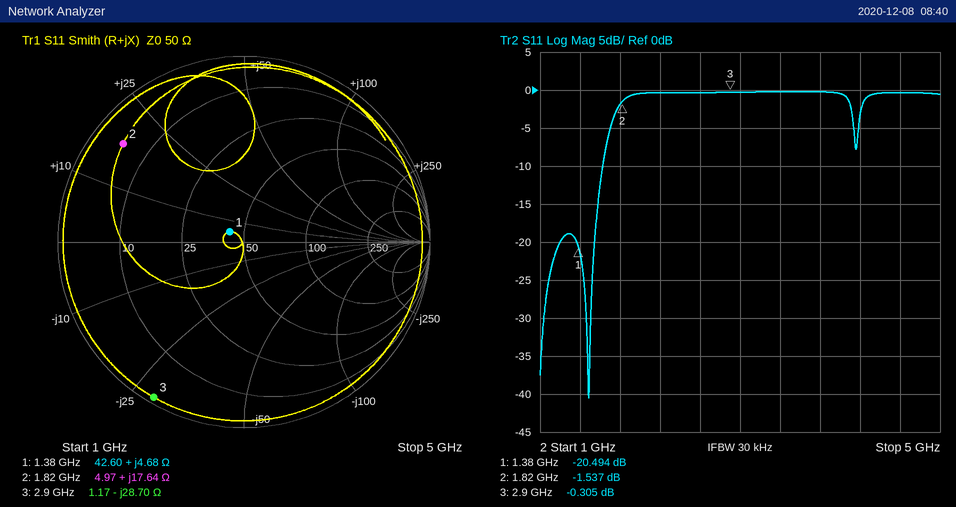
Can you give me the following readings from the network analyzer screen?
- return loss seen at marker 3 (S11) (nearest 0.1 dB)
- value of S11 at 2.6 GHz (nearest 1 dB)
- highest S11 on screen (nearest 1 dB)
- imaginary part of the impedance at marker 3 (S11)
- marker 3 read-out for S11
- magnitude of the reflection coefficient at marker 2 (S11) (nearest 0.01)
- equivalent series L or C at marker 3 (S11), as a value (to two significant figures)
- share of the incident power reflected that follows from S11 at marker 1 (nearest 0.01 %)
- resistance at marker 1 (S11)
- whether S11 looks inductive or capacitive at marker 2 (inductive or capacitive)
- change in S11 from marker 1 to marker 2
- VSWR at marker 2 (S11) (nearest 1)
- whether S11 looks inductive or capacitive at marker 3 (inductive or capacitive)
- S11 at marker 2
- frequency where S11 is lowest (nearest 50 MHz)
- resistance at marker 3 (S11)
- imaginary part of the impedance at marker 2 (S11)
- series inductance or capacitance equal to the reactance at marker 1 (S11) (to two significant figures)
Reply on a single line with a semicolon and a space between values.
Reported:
0.3 dB; 0 dB; 0 dB; -28.70 Ω; -0.305 dB; 0.84; 1.9 pF; 0.89 %; 42.60 Ω; inductive; 18.957 dB; 11; capacitive; -1.537 dB; 1.50 GHz; 1.17 Ω; +17.64 Ω; 540 pH
